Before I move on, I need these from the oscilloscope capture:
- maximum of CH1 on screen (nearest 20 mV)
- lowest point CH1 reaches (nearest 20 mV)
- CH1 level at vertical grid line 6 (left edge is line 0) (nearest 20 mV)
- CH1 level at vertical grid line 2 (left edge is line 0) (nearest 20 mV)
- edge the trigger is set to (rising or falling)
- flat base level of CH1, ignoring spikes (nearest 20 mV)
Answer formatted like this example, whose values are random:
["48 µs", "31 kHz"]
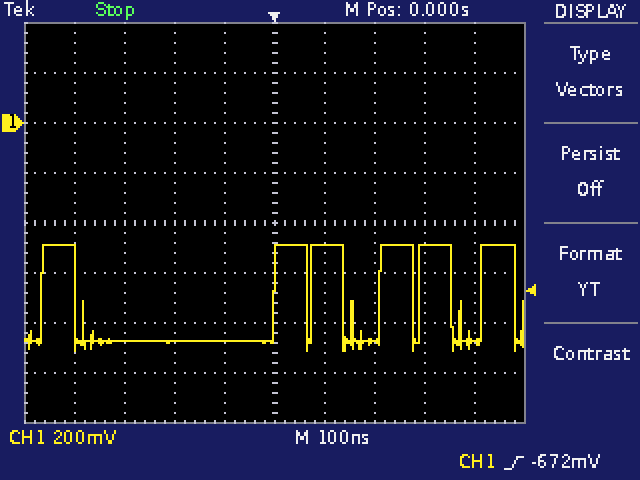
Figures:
["-480 mV", "-920 mV", "-480 mV", "-880 mV", "rising", "-880 mV"]
